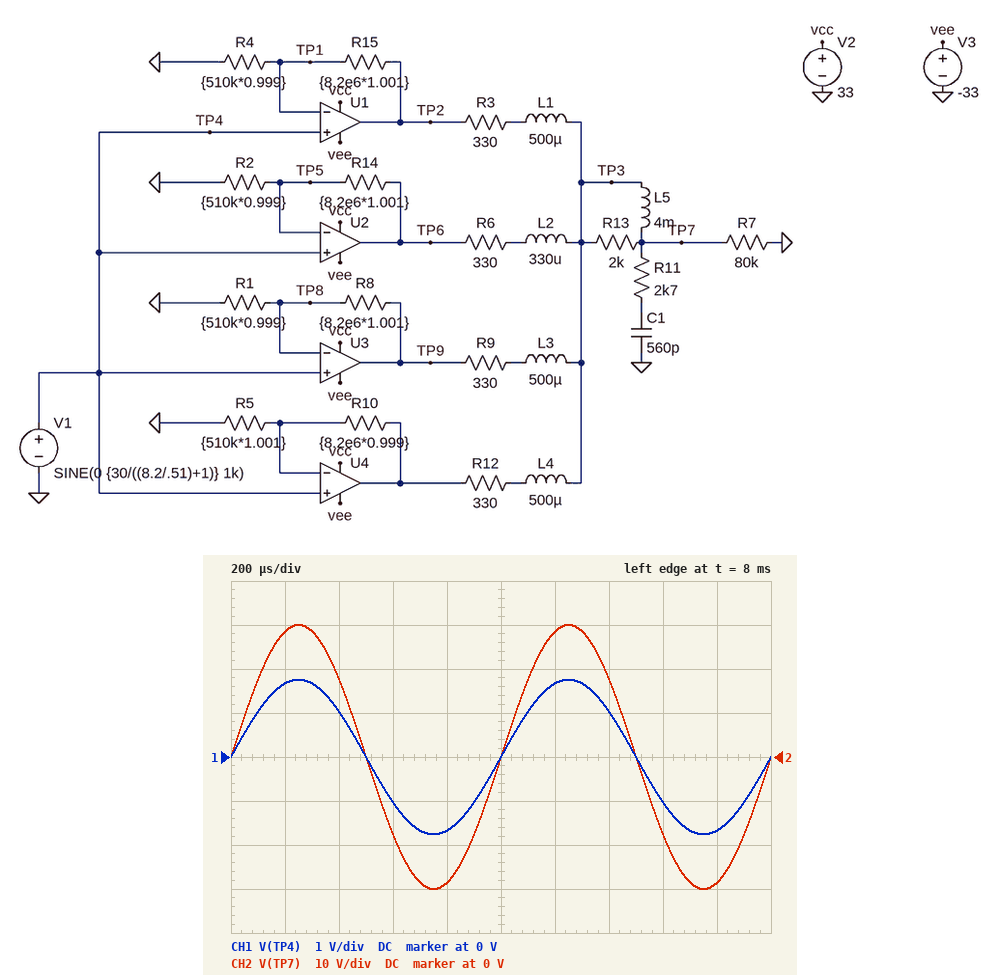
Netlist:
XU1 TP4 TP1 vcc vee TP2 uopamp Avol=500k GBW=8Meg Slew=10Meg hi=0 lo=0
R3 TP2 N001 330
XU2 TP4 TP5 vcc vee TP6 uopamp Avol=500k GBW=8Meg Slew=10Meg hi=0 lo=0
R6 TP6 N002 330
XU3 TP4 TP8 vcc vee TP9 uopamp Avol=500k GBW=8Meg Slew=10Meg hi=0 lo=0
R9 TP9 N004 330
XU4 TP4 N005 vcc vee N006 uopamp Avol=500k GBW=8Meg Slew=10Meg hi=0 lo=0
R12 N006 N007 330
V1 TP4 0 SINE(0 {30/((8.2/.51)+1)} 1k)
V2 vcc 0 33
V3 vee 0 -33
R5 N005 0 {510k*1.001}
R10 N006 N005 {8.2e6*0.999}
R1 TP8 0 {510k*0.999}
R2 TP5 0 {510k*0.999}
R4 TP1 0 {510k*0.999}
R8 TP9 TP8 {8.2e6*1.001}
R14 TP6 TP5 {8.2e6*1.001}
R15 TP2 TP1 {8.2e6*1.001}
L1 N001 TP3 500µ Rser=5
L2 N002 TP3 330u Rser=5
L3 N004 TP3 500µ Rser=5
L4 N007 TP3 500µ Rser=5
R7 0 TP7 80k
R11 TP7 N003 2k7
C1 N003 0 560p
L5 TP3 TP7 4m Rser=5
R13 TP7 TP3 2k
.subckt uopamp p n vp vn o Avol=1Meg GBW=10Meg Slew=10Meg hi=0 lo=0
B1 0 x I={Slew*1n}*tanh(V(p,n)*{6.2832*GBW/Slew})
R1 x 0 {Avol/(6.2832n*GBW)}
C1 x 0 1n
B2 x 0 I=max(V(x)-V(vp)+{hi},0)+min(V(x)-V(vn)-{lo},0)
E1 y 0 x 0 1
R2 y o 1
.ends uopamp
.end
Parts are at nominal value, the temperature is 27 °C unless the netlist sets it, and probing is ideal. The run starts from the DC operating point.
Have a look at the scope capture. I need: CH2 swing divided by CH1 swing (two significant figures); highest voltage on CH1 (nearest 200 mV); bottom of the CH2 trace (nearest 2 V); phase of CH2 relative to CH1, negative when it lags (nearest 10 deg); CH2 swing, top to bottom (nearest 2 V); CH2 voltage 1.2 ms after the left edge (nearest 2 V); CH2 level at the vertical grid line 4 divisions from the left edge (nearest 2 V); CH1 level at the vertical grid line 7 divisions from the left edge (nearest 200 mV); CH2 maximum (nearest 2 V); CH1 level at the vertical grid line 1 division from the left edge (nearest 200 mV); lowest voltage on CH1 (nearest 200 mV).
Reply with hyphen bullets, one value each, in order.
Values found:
- 17
- 1.8 V
- -30 V
- 0 deg
- 60 V
- 28 V
- -28 V
- 1.0 V
- 30 V
- 1.6 V
- -1.8 V
